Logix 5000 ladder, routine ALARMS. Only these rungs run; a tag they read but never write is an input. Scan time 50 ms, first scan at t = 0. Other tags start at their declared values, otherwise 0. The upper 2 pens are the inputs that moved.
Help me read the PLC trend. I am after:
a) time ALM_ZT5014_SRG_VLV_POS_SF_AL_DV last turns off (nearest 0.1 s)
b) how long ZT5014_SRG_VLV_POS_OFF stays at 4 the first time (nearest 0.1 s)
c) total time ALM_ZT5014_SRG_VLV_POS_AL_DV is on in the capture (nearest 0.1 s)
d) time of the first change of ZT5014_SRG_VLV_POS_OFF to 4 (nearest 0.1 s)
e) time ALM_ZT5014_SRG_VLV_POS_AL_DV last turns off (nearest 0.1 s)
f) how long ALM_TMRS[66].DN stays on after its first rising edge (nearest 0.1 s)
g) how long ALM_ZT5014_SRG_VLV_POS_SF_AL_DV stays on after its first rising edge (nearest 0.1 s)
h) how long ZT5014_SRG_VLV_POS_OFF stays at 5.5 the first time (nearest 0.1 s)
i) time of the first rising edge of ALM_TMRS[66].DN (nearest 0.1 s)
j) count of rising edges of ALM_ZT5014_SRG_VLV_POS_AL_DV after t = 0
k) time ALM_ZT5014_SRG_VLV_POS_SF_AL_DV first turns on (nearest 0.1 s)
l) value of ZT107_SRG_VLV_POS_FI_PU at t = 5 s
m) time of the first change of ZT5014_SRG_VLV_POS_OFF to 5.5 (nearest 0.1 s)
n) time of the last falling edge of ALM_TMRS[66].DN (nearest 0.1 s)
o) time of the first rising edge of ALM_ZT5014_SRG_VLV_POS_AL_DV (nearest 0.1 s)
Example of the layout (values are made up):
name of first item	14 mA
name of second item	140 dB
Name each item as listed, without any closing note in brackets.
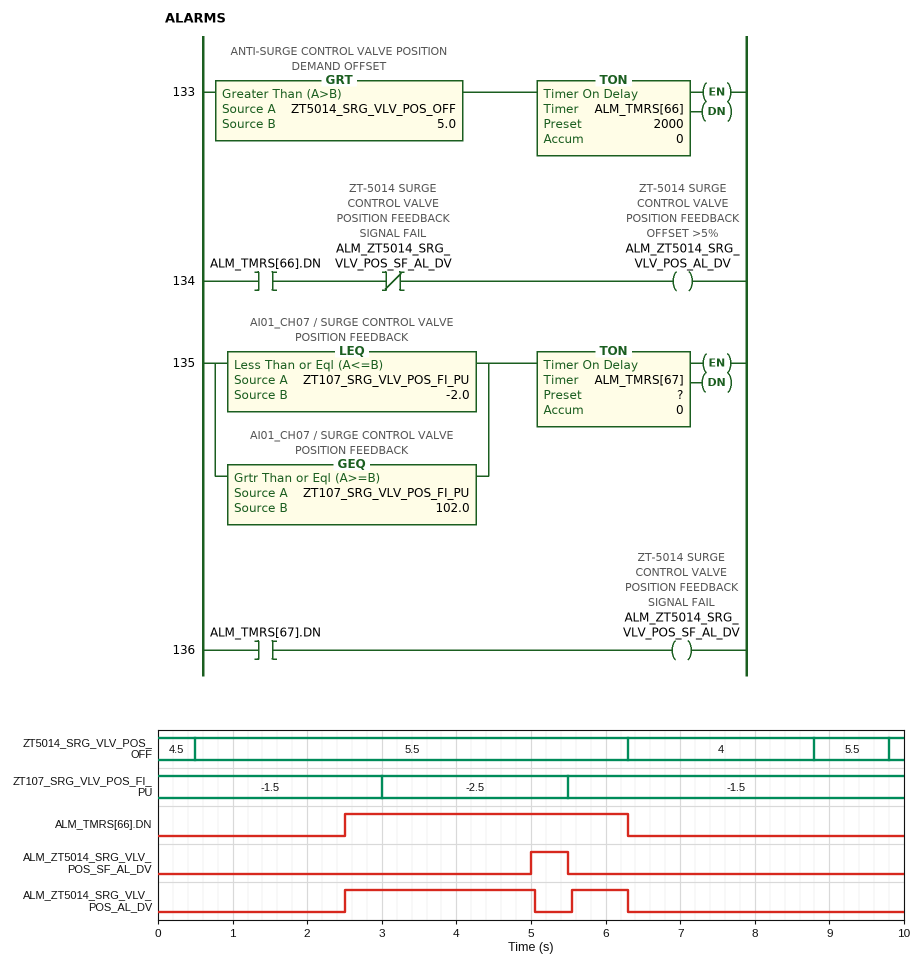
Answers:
time ALM_ZT5014_SRG_VLV_POS_SF_AL_DV last turns off	5.5 s
how long ZT5014_SRG_VLV_POS_OFF stays at 4 the first time	2.5 s
total time ALM_ZT5014_SRG_VLV_POS_AL_DV is on in the capture	3.3 s
time of the first change of ZT5014_SRG_VLV_POS_OFF to 4	6.3 s
time ALM_ZT5014_SRG_VLV_POS_AL_DV last turns off	6.3 s
how long ALM_TMRS[66].DN stays on after its first rising edge	3.8 s
how long ALM_ZT5014_SRG_VLV_POS_SF_AL_DV stays on after its first rising edge	0.5 s
how long ZT5014_SRG_VLV_POS_OFF stays at 5.5 the first time	5.8 s
time of the first rising edge of ALM_TMRS[66].DN	2.5 s
count of rising edges of ALM_ZT5014_SRG_VLV_POS_AL_DV after t = 0	2
time ALM_ZT5014_SRG_VLV_POS_SF_AL_DV first turns on	5.0 s
value of ZT107_SRG_VLV_POS_FI_PU at t = 5 s	-2.5
time of the first change of ZT5014_SRG_VLV_POS_OFF to 5.5	0.5 s
time of the last falling edge of ALM_TMRS[66].DN	6.3 s
time of the first rising edge of ALM_ZT5014_SRG_VLV_POS_AL_DV	2.5 s
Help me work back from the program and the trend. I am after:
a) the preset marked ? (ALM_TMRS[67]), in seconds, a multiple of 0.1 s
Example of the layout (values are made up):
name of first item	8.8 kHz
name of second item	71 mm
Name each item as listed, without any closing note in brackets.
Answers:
the preset marked ? (ALM_TMRS[67]), in seconds, a multiple of 0.1 s	2.0 s
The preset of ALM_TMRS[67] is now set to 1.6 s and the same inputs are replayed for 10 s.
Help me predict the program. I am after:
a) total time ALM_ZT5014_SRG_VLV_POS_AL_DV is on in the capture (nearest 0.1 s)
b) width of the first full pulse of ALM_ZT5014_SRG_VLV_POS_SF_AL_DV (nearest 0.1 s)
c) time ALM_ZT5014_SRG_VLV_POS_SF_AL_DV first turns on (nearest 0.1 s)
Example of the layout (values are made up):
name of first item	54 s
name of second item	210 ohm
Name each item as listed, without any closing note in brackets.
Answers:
total time ALM_ZT5014_SRG_VLV_POS_AL_DV is on in the capture	2.9 s
width of the first full pulse of ALM_ZT5014_SRG_VLV_POS_SF_AL_DV	0.9 s
time ALM_ZT5014_SRG_VLV_POS_SF_AL_DV first turns on	4.6 s
